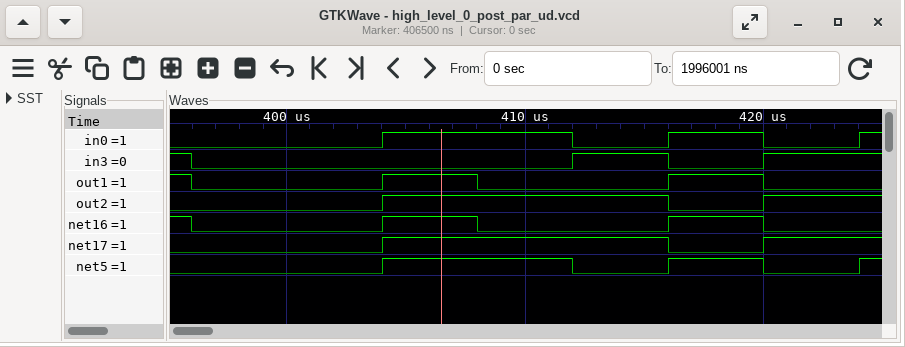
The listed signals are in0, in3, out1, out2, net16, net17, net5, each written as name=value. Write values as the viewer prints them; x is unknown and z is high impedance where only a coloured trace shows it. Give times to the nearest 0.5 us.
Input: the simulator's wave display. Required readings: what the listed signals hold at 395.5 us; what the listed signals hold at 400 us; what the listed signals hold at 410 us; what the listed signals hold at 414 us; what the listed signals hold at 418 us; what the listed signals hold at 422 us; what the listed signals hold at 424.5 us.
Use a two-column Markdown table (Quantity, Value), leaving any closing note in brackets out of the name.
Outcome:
| Quantity | Value |
|---|---|
| what the listed signals hold at 395.5 us | in0=0, in3=1, out1=1, out2=0, net16=1, net17=0, net5=0 |
| what the listed signals hold at 400 us | in0=0, in3=0, out1=0, out2=0, net16=0, net17=0, net5=0 |
| what the listed signals hold at 410 us | in0=1, in3=0, out1=0, out2=1, net16=0, net17=1, net5=1 |
| what the listed signals hold at 414 us | in0=0, in3=1, out1=0, out2=1, net16=0, net17=1, net5=0 |
| what the listed signals hold at 418 us | in0=1, in3=0, out1=1, out2=0, net16=1, net17=0, net5=1 |
| what the listed signals hold at 422 us | in0=0, in3=1, out1=0, out2=1, net16=0, net17=1, net5=0 |
| what the listed signals hold at 424.5 us | in0=1, in3=1, out1=0, out2=1, net16=0, net17=1, net5=1 |
